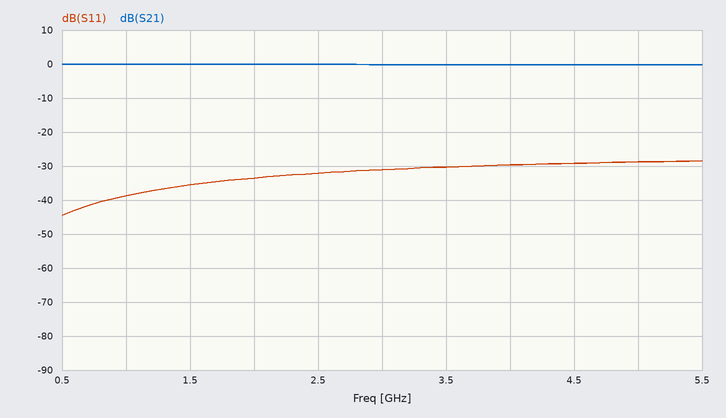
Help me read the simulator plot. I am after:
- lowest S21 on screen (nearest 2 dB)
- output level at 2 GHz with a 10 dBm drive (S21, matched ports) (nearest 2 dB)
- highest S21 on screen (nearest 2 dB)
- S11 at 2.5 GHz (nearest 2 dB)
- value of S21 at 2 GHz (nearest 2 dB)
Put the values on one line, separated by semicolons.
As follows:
0 dB; 10 dBm; 0 dB; -32 dB; 0 dB
